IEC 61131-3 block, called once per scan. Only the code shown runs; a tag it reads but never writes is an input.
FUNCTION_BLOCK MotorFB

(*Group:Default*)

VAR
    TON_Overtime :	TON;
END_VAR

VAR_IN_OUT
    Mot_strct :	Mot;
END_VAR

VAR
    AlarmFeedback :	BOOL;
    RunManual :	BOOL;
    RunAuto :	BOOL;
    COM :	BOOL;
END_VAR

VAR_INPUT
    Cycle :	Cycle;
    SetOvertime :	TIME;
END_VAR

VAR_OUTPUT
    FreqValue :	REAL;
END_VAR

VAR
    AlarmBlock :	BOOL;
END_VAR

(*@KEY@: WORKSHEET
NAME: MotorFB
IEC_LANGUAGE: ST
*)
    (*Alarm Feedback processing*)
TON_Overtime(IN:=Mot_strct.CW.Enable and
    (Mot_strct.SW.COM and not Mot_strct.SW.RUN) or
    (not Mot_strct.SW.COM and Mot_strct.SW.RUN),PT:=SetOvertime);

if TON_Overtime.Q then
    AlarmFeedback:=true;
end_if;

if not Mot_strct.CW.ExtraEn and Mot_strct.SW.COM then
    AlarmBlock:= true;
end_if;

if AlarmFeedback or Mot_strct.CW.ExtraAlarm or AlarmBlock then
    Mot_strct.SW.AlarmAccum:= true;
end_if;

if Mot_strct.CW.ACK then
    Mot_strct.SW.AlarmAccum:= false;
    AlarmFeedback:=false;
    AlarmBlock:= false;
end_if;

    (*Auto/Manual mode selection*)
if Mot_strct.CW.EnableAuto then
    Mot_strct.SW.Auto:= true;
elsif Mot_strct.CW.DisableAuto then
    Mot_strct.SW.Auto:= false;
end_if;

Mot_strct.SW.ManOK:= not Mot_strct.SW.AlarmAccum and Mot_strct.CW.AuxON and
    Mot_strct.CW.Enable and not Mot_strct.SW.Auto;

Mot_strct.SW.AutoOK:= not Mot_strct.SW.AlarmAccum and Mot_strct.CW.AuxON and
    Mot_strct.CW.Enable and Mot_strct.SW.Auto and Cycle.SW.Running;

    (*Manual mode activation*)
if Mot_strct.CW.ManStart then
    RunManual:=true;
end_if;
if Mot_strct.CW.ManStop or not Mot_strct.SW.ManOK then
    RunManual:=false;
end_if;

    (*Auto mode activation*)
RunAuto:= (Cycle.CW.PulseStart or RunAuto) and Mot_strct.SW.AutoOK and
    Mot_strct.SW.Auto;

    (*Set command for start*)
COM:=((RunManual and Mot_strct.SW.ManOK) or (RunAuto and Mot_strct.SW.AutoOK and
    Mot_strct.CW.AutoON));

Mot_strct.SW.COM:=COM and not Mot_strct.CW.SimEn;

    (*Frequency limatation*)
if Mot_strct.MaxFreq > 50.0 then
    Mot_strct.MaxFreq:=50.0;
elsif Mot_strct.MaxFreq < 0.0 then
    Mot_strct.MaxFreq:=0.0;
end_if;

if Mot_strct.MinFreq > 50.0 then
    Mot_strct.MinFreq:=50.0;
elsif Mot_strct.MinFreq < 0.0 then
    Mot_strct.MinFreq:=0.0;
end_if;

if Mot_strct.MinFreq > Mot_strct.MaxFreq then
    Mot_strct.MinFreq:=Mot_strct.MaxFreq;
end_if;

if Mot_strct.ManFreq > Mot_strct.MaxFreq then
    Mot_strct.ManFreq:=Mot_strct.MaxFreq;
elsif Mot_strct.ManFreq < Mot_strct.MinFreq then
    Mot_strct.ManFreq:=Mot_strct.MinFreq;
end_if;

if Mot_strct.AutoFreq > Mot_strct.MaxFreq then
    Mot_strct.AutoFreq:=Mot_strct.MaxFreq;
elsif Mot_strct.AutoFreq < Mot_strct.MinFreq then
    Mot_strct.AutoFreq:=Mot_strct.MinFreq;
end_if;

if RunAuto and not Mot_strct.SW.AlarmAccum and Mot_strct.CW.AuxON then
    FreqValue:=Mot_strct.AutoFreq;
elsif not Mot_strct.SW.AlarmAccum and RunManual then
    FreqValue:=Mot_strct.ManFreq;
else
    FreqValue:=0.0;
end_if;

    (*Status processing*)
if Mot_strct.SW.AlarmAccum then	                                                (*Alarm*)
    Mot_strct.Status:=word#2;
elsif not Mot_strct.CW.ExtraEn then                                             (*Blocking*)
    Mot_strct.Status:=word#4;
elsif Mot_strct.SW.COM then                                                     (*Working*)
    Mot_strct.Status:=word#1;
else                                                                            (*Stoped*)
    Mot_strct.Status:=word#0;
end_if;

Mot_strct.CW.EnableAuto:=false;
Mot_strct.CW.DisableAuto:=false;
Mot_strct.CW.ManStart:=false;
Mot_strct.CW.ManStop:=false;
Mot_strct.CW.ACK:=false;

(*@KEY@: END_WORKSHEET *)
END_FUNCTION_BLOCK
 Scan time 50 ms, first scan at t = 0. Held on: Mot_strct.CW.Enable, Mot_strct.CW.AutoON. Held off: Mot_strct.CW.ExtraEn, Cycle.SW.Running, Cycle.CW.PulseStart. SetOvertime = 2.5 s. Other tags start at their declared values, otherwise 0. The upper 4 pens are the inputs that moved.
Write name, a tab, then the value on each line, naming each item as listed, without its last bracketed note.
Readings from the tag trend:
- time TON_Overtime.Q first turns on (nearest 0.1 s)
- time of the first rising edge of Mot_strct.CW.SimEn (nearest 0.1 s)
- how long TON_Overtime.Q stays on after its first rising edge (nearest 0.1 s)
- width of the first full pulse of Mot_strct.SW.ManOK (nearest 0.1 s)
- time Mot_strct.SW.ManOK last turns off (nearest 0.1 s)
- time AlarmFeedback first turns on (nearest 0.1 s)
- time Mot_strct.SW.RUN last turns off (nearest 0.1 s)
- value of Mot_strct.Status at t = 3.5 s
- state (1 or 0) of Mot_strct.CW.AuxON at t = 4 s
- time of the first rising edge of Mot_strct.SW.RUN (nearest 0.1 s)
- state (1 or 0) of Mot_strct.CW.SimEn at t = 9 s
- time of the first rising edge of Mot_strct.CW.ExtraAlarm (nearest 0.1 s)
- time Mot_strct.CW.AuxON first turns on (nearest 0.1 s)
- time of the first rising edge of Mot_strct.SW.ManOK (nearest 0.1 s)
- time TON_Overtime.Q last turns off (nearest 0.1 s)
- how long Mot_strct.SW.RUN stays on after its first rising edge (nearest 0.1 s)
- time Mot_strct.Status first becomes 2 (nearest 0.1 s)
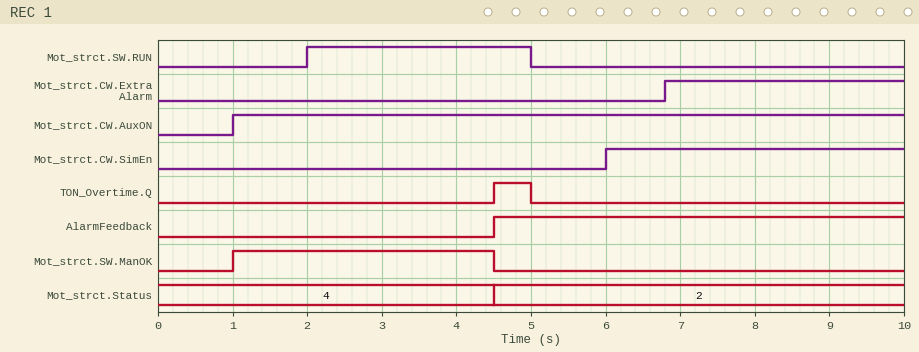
time TON_Overtime.Q first turns on	4.5 s
time of the first rising edge of Mot_strct.CW.SimEn	6.0 s
how long TON_Overtime.Q stays on after its first rising edge	0.5 s
width of the first full pulse of Mot_strct.SW.ManOK	3.5 s
time Mot_strct.SW.ManOK last turns off	4.5 s
time AlarmFeedback first turns on	4.5 s
time Mot_strct.SW.RUN last turns off	5.0 s
value of Mot_strct.Status at t = 3.5 s	4
state (1 or 0) of Mot_strct.CW.AuxON at t = 4 s	1
time of the first rising edge of Mot_strct.SW.RUN	2.0 s
state (1 or 0) of Mot_strct.CW.SimEn at t = 9 s	1
time of the first rising edge of Mot_strct.CW.ExtraAlarm	6.8 s
time Mot_strct.CW.AuxON first turns on	1.0 s
time of the first rising edge of Mot_strct.SW.ManOK	1.0 s
time TON_Overtime.Q last turns off	5.0 s
how long Mot_strct.SW.RUN stays on after its first rising edge	3.0 s
time Mot_strct.Status first becomes 2	4.5 s
